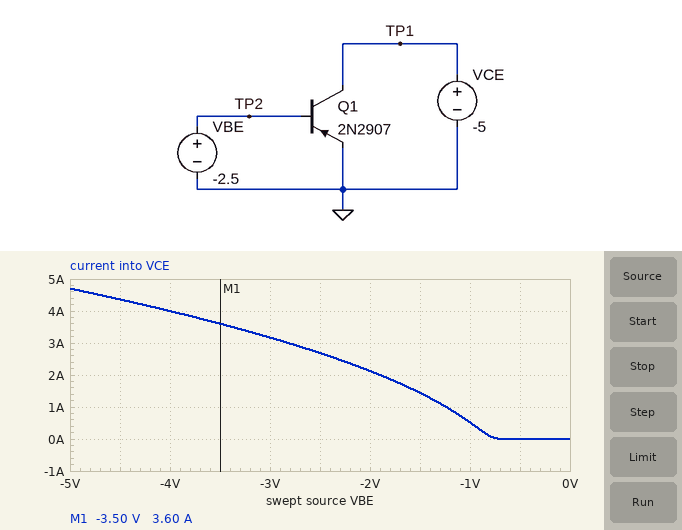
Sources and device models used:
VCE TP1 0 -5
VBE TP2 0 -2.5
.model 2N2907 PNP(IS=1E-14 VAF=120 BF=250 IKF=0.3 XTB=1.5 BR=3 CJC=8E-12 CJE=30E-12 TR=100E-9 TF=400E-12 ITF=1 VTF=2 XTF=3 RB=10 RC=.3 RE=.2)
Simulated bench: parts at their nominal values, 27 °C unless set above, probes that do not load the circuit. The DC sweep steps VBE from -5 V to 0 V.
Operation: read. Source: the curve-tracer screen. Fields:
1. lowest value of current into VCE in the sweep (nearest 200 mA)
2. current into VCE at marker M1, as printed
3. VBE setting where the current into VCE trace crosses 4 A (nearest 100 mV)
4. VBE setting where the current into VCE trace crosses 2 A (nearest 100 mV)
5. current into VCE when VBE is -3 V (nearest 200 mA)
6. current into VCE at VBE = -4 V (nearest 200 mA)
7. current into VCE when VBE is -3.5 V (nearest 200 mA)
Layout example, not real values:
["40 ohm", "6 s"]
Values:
["0 A", "3.60 A", "-4.0 V", "-1.9 V", "3.2 A", "4.0 A", "3.6 A"]
